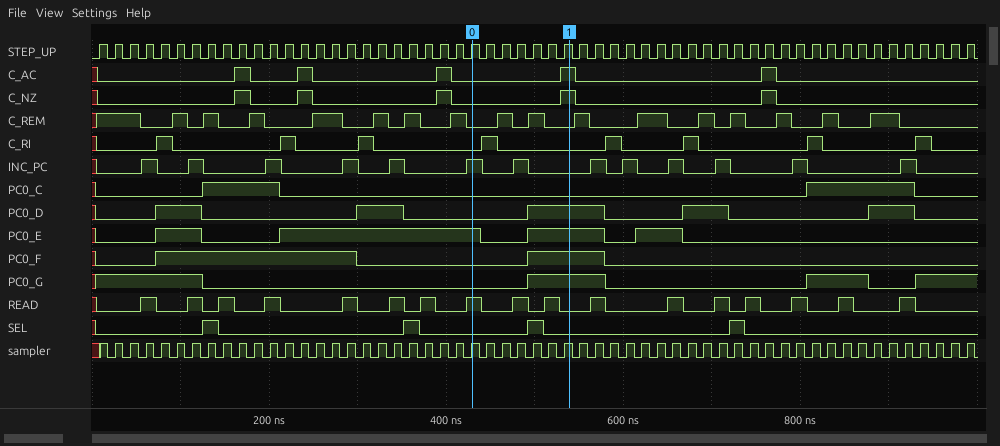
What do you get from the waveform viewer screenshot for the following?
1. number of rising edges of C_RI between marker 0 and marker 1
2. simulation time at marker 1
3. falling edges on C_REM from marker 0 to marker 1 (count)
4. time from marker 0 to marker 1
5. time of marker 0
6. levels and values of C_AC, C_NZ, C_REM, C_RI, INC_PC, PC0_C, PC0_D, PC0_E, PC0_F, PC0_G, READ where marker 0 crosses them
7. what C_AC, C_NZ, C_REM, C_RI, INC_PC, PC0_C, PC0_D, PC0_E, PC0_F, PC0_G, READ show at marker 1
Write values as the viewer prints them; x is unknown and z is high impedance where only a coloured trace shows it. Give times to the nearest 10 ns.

1
540 ns
2
110 ns
430 ns
C_AC=0, C_NZ=0, C_REM=0, C_RI=0, INC_PC=1, PC0_C=0, PC0_D=0, PC0_E=1, PC0_F=0, PC0_G=0, READ=1
C_AC=1, C_NZ=1, C_REM=0, C_RI=0, INC_PC=0, PC0_C=0, PC0_D=1, PC0_E=1, PC0_F=1, PC0_G=1, READ=0
